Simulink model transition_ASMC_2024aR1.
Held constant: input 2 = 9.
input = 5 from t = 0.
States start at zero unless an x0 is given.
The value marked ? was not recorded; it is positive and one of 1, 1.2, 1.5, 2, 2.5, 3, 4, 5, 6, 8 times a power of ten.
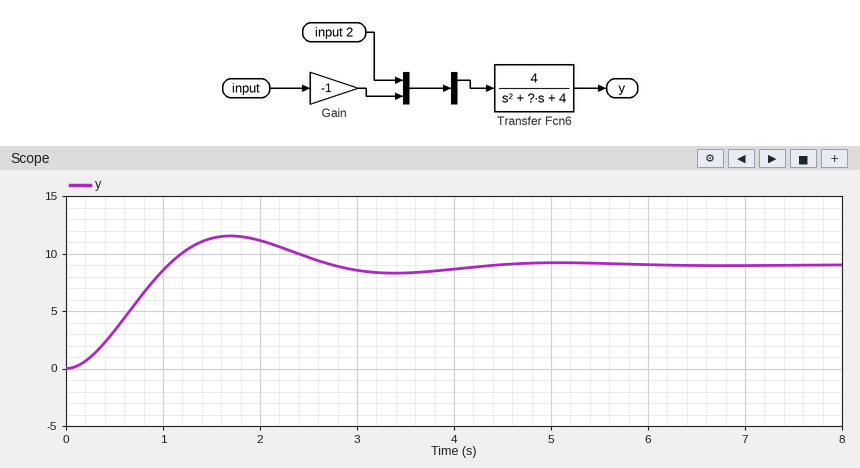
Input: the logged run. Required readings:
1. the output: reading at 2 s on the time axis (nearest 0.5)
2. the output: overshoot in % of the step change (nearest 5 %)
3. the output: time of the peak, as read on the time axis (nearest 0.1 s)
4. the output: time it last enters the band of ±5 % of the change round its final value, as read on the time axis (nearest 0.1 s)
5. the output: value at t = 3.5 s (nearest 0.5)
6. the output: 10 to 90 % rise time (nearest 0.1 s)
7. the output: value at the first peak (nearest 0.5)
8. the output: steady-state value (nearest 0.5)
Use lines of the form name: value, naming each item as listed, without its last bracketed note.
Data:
the output: reading at 2 s on the time axis: 11.0
the output: overshoot in % of the step change: 30 %
the output: time of the peak, as read on the time axis: 1.7 s
the output: time it last enters the band of ±5 % of the change round its final value, as read on the time axis: 3.9 s
the output: value at t = 3.5 s: 8.5
the output: 10 to 90 % rise time: 0.7 s
the output: value at the first peak: 11.5
the output: steady-state value: 9.0
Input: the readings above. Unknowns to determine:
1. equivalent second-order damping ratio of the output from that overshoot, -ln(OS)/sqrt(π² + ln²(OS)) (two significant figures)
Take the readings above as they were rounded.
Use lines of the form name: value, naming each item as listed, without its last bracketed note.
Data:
equivalent second-order damping ratio of the output from that overshoot, -ln(OS)/sqrt(π² + ln²(OS)): 0.36
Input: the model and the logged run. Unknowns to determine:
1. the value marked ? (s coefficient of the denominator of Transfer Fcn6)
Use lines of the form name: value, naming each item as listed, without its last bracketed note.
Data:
the value marked ?: 1.5
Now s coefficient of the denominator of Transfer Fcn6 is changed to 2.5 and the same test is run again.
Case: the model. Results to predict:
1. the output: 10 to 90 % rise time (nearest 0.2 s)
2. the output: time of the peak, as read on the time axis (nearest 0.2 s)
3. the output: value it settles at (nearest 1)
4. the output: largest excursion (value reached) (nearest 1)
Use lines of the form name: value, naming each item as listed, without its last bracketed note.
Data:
the output: 10 to 90 % rise time: 1.0 s
the output: time of the peak, as read on the time axis: 2.0 s
the output: value it settles at: 9
the output: largest excursion (value reached): 10
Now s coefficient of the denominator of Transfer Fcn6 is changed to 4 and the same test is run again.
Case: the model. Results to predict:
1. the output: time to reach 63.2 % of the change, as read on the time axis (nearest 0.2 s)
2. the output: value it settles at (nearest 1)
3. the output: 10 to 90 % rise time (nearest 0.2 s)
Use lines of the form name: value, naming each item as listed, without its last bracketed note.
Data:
the output: time to reach 63.2 % of the change, as read on the time axis: 1.0 s
the output: value it settles at: 9
the output: 10 to 90 % rise time: 1.6 s
